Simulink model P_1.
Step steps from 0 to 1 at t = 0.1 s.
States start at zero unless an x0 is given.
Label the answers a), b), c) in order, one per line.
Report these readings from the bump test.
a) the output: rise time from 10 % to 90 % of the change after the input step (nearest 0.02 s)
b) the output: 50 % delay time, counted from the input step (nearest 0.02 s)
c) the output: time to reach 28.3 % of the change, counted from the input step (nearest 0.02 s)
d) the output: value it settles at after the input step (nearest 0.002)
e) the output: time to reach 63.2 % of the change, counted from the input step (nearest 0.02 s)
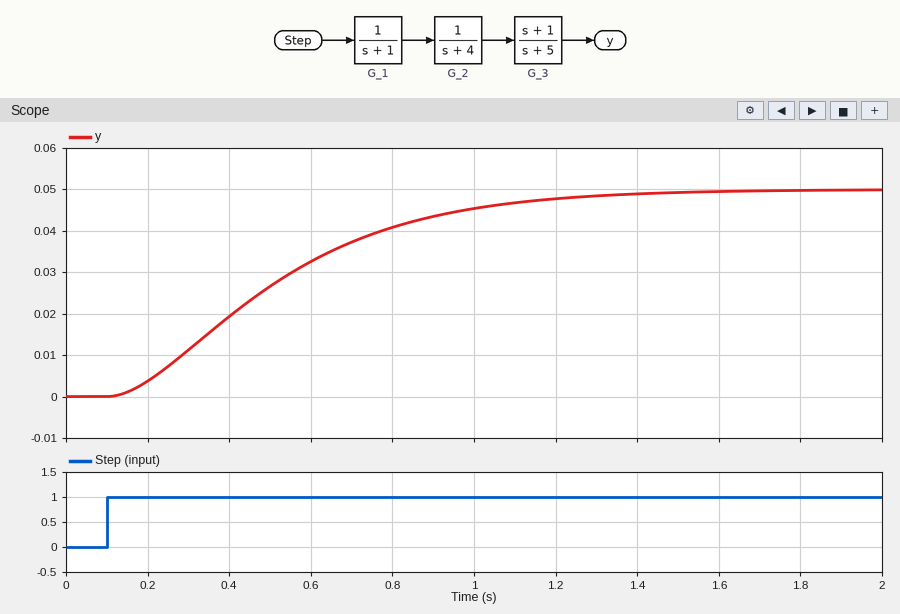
a) 0.76 s
b) 0.38 s
c) 0.24 s
d) 0.050
e) 0.48 s
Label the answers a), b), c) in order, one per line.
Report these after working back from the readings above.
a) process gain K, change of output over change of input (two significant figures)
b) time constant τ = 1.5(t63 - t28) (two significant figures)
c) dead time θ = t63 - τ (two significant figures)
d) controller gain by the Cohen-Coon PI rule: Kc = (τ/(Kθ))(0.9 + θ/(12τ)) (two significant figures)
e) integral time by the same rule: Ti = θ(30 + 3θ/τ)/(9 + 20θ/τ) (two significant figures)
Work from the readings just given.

a) 0.050
b) 0.36 s
c) 0.12 s
d) 56
e) 0.24 s
